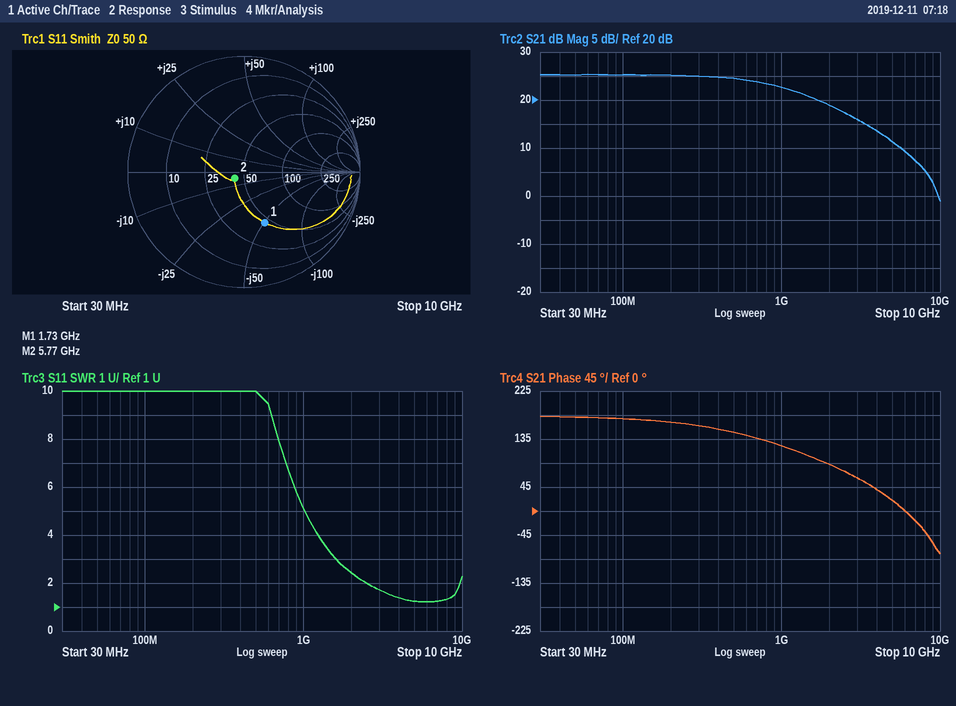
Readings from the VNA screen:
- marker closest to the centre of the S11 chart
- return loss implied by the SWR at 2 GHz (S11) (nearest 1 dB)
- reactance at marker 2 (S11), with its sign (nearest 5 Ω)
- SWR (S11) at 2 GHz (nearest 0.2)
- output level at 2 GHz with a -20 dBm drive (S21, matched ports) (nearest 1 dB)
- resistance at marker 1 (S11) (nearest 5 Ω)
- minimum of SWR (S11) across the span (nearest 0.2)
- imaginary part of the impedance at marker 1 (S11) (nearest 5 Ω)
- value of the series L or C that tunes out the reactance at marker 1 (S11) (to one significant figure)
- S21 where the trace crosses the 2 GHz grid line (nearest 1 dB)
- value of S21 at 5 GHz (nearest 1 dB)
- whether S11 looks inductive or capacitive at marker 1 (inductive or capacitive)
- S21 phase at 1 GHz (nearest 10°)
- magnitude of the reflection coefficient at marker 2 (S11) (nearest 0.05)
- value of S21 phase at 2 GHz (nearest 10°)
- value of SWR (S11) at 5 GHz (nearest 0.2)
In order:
marker 2
8 dB
-5 Ω
2.4
-1 dBm
45 Ω
1.2
-50 Ω
5 nH
19 dB
11 dB
capacitive
120°
0.10
90°
1.2
